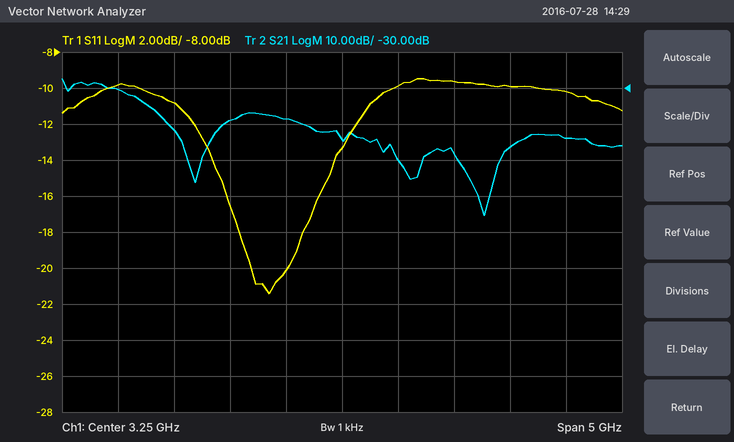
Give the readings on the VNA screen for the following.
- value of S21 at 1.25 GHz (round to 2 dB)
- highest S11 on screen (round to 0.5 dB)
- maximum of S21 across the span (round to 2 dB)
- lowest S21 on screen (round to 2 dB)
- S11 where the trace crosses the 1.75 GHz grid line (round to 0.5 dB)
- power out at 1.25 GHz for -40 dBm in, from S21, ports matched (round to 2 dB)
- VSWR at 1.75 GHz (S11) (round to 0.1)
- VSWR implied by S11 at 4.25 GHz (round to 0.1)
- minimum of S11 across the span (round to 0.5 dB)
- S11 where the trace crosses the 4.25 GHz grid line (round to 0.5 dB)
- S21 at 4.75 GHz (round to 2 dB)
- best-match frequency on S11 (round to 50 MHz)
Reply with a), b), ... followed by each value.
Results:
a) -30 dB
b) -9.5 dB
c) -28 dB
d) -66 dB
e) -11.0 dB
f) -70 dBm
g) 1.8
h) 2.0
i) -21.5 dB
j) -9.5 dB
k) -46 dB
l) 2.60 GHz
